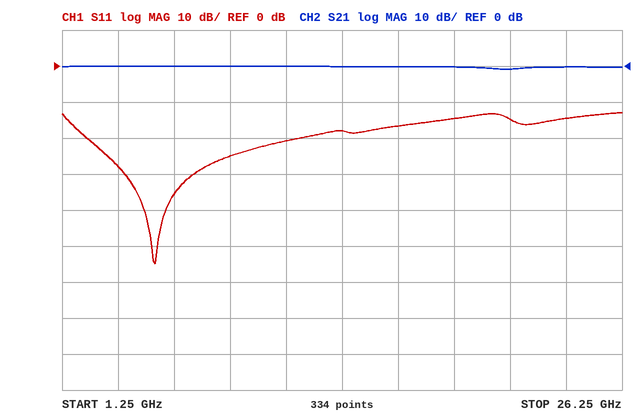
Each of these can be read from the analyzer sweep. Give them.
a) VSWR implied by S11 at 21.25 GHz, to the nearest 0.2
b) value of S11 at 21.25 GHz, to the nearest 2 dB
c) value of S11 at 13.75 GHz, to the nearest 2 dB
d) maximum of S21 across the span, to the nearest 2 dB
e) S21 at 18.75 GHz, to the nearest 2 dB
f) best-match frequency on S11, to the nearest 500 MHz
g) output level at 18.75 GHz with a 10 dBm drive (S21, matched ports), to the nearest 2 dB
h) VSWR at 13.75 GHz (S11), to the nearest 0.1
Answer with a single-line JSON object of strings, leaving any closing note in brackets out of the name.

{"VSWR implied by S11 at 21.25 GHz, to the nearest 0.2": "1.4", "value of S11 at 21.25 GHz, to the nearest 2 dB": "-14 dB", "value of S11 at 13.75 GHz, to the nearest 2 dB": "-18 dB", "maximum of S21 across the span, to the nearest 2 dB": "0 dB", "S21 at 18.75 GHz, to the nearest 2 dB": "0 dB", "best-match frequency on S11, to the nearest 500 MHz": "5.5 GHz", "output level at 18.75 GHz with a 10 dBm drive (S21, matched ports), to the nearest 2 dB": "10 dBm", "VSWR at 13.75 GHz (S11), to the nearest 0.1": "1.3"}
